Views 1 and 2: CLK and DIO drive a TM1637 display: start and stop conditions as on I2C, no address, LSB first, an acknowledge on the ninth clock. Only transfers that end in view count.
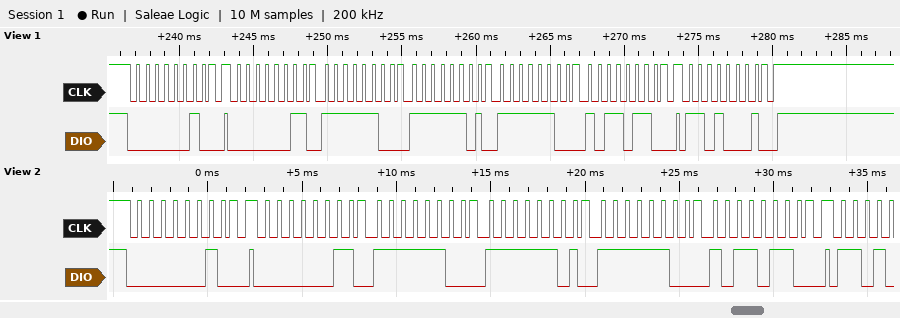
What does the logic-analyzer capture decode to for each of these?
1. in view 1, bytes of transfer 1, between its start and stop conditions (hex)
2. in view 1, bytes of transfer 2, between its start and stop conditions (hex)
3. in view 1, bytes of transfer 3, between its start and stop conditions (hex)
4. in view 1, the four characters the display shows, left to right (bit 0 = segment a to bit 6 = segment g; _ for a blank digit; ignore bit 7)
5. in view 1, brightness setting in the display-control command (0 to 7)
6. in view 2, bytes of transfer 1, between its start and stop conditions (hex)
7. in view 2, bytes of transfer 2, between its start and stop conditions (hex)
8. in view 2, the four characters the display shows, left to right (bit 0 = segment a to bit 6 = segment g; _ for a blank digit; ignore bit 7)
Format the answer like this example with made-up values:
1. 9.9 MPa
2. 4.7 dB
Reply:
1. 40
2. C0 3F BF 3F 6D
3. 8B
4. 0005
5. 3
6. 40
7. C0 3F BF 3F 6D
8. 0005
